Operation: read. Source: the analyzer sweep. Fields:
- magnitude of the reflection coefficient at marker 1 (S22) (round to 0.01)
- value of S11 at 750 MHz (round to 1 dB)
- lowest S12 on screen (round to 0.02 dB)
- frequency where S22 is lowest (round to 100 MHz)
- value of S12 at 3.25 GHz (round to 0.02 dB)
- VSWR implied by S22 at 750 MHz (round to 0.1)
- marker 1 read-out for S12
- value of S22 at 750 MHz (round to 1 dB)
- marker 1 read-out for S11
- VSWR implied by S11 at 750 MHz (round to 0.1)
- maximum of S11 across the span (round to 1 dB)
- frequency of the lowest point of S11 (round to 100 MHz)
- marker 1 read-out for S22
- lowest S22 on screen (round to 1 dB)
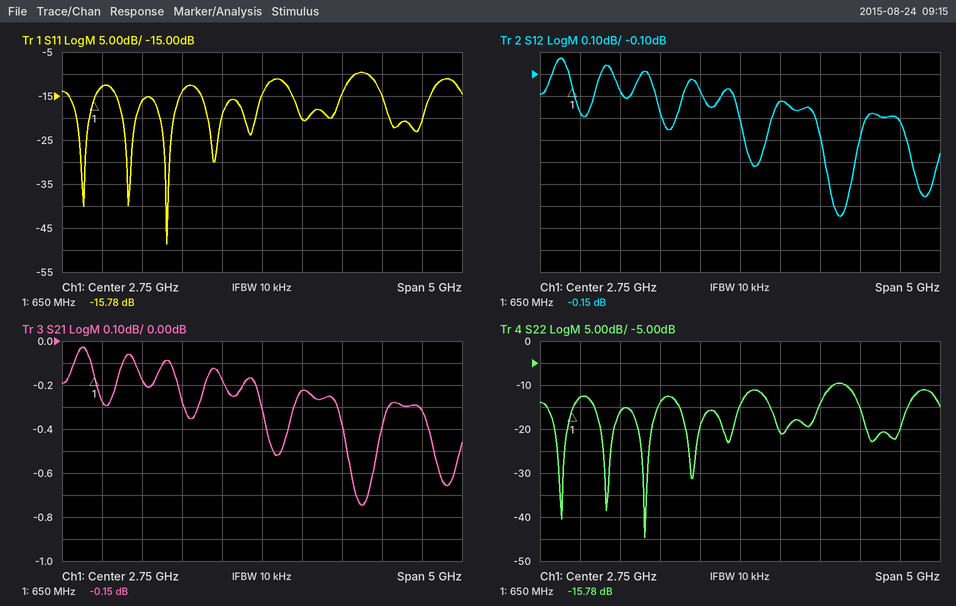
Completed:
0.16
-13 dB
-0.74 dB
1.6 GHz
-0.22 dB
1.6
-0.15 dB
-13 dB
-15.78 dB
1.6
-10 dB
1.6 GHz
-15.78 dB
-45 dB
